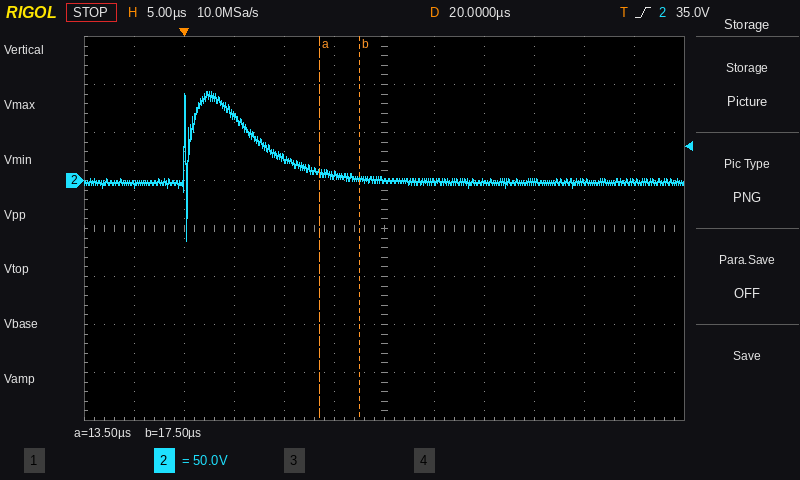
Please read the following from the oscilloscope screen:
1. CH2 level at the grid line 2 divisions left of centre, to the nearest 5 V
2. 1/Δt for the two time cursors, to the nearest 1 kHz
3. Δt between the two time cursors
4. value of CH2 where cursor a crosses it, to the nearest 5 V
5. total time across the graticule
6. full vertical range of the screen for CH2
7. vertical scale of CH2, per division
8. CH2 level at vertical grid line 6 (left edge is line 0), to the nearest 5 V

25 V
250 kHz
4.0 µs
10 V
60 µs
400 V
50 V
0 V
